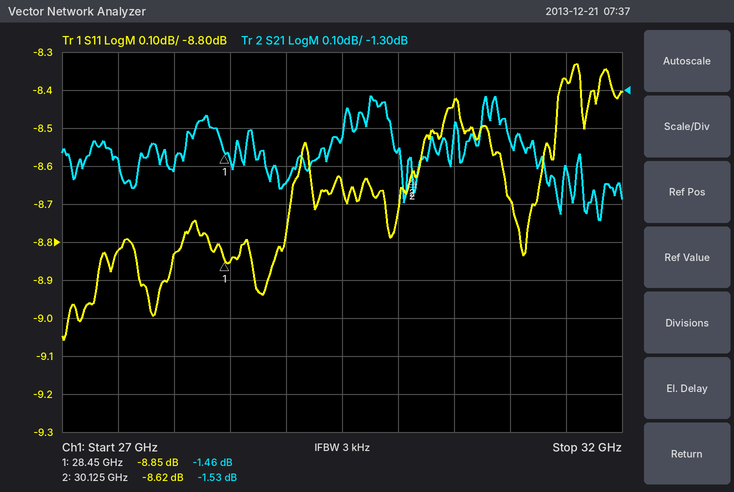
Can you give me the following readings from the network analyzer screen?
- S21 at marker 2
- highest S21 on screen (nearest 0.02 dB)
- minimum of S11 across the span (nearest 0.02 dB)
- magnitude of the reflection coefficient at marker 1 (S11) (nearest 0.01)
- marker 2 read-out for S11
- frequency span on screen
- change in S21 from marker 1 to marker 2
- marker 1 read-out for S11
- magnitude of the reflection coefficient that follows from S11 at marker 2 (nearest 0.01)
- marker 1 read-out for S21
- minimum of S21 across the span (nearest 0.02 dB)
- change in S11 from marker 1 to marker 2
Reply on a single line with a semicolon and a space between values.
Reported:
-1.53 dB; -1.32 dB; -9.06 dB; 0.36; -8.62 dB; 5 GHz; -0.07 dB; -8.85 dB; 0.37; -1.46 dB; -1.64 dB; 0.23 dB
